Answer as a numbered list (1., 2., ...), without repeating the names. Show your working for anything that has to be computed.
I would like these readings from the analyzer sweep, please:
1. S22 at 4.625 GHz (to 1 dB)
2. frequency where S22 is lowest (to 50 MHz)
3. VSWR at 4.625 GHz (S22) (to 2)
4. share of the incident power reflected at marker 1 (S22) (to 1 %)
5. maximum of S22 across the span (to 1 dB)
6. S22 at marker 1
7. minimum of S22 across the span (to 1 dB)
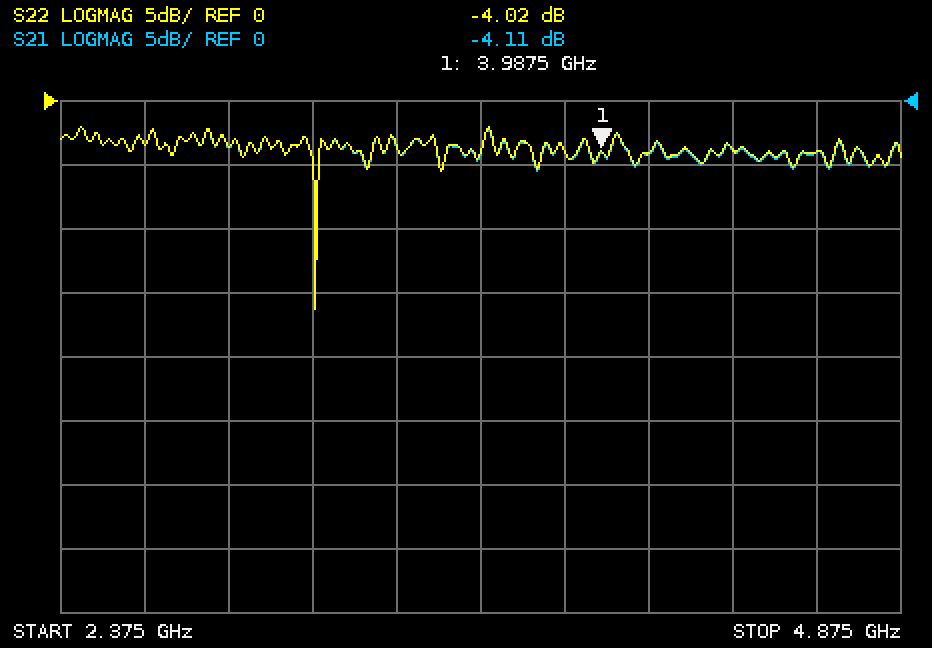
1. -4 dB
2. 3.15 GHz
3. |Γ| = 10^(-4/20) = 0.6310; VSWR = (1 + 0.6310)/(1 − 0.6310) ≈ 4
4. 10^(-4.02/10) ≈ 40 %
5. -2 dB
6. -4.02 dB
7. -16 dB
